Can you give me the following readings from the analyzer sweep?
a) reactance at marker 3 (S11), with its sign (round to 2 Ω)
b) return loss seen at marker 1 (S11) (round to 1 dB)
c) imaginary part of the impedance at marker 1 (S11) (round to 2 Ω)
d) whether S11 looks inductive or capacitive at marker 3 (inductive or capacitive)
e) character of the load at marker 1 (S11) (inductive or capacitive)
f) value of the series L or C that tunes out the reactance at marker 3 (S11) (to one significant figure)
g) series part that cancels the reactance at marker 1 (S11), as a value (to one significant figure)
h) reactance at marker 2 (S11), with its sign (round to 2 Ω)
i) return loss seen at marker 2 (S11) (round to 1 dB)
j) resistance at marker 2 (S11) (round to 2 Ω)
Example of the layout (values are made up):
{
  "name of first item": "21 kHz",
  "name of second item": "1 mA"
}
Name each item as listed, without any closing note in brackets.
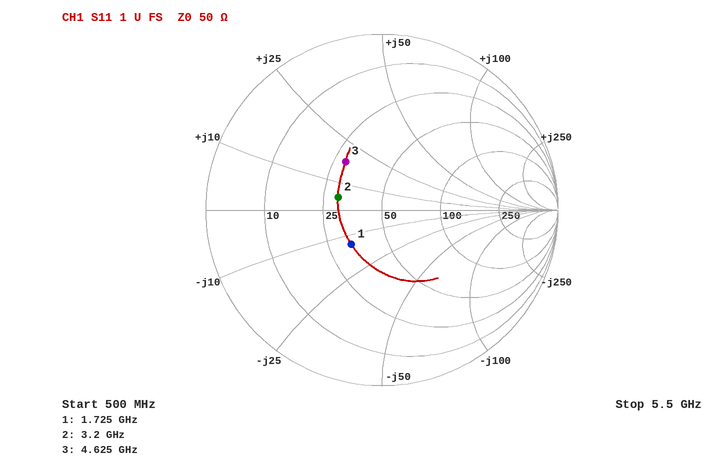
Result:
{
  "reactance at marker 3 (S11), with its sign": "+18 Ω",
  "return loss seen at marker 1 (S11)": "12 dB",
  "imaginary part of the impedance at marker 1 (S11)": "-14 Ω",
  "whether S11 looks inductive or capacitive at marker 3": "inductive",
  "character of the load at marker 1 (S11)": "capacitive",
  "value of the series L or C that tunes out the reactance at marker 3 (S11)": "2 pF",
  "series part that cancels the reactance at marker 1 (S11), as a value": "1 nH",
  "reactance at marker 2 (S11), with its sign": "+4 Ω",
  "return loss seen at marker 2 (S11)": "12 dB",
  "resistance at marker 2 (S11)": "30 Ω"
}
